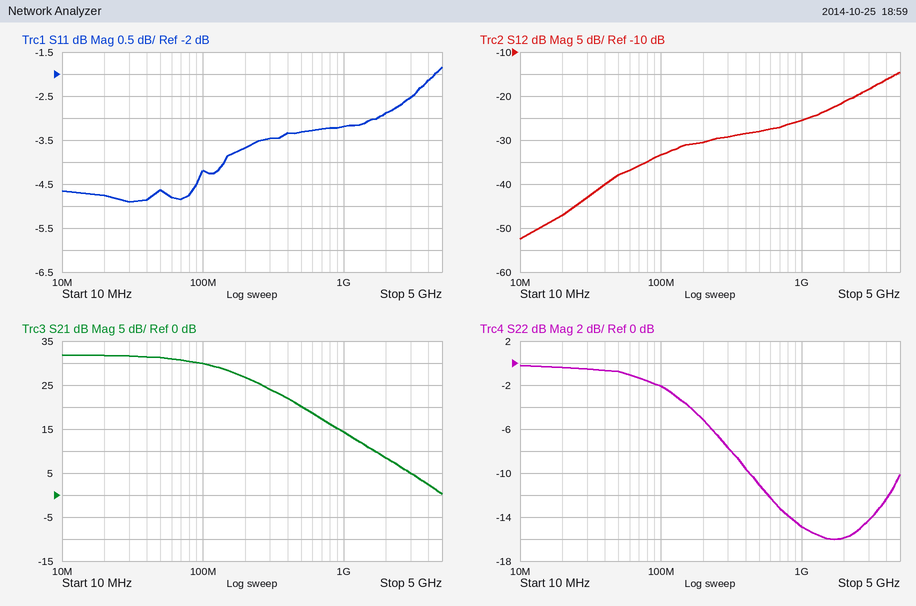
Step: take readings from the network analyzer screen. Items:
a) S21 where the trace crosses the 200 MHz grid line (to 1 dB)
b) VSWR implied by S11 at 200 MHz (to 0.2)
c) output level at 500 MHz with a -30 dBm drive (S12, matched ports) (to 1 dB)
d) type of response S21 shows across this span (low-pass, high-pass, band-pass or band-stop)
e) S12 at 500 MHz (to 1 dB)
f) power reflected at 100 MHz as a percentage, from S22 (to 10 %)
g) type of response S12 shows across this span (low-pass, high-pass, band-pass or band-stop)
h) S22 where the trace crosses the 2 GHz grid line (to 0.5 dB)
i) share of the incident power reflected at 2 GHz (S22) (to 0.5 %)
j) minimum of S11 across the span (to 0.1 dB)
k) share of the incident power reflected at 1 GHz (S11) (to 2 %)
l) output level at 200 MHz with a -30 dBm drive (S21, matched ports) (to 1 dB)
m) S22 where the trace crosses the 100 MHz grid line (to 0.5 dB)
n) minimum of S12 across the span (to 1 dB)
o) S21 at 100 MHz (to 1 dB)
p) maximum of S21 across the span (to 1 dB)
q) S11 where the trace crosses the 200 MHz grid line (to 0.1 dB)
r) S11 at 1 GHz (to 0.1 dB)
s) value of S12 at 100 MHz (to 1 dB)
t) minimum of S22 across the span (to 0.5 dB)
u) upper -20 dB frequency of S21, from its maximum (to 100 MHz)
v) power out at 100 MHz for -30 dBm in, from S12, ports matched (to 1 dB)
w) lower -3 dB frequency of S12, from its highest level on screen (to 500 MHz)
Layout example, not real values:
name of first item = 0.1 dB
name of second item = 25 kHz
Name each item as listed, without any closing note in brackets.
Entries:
S21 where the trace crosses the 200 MHz grid line = 27 dB
VSWR implied by S11 at 200 MHz = 4.8
output level at 500 MHz with a -30 dBm drive (S12, matched ports) = -58 dBm
type of response S21 shows across this span = low-pass
S12 at 500 MHz = -28 dB
power reflected at 100 MHz as a percentage, from S22 = 60 %
type of response S12 shows across this span = high-pass
S22 where the trace crosses the 2 GHz grid line = -16.0 dB
share of the incident power reflected at 2 GHz (S22) = 2.5 %
minimum of S11 across the span = -4.9 dB
share of the incident power reflected at 1 GHz (S11) = 48 %
output level at 200 MHz with a -30 dBm drive (S21, matched ports) = -3 dBm
S22 where the trace crosses the 100 MHz grid line = -2.0 dB
minimum of S12 across the span = -52 dB
S21 at 100 MHz = 30 dB
maximum of S21 across the span = 32 dB
S11 where the trace crosses the 200 MHz grid line = -3.7 dB
S11 at 1 GHz = -3.2 dB
value of S12 at 100 MHz = -33 dB
minimum of S22 across the span = -16.0 dB
upper -20 dB frequency of S21, from its maximum = 1.3 GHz
power out at 100 MHz for -30 dBm in, from S12, ports matched = -63 dBm
lower -3 dB frequency of S12, from its highest level on screen = 3.5 GHz
